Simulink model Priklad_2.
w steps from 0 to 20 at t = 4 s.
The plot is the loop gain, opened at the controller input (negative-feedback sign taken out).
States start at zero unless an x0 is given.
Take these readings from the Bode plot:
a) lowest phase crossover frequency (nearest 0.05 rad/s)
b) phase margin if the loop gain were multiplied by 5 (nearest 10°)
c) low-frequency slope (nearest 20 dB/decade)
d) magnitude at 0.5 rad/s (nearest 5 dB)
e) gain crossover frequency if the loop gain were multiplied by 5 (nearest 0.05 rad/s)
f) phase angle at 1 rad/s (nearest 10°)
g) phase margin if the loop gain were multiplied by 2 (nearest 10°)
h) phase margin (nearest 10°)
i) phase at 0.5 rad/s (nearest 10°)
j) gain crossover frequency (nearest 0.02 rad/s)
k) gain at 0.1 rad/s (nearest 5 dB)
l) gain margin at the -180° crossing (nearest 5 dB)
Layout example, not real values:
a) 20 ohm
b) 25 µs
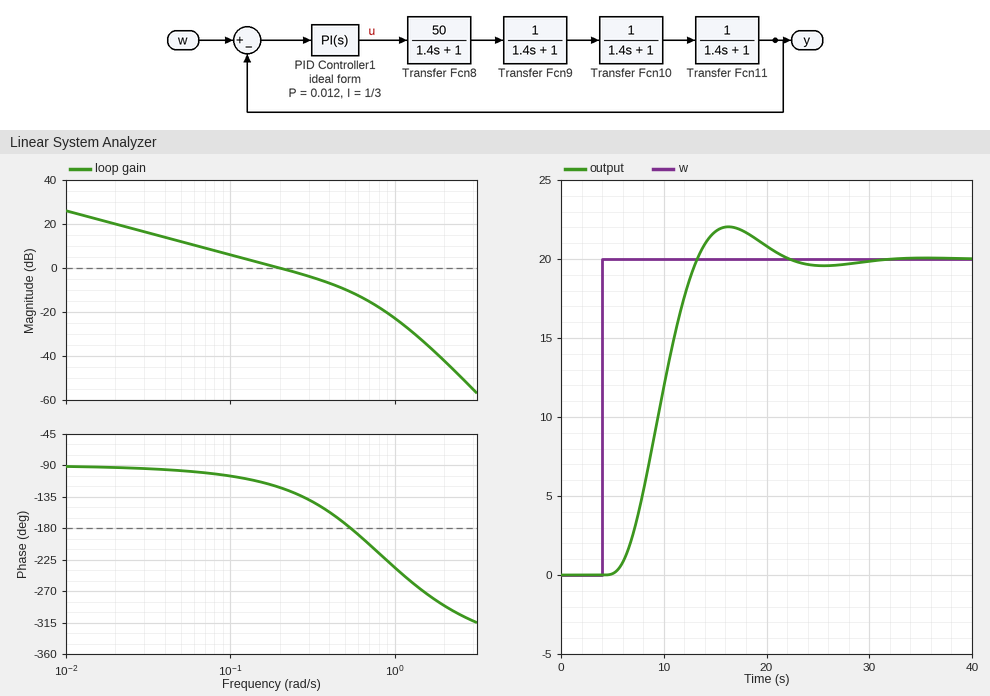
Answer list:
a) 0.55 rad/s
b) -20°
c) -20 dB/decade
d) -10 dB
e) 0.65 rad/s
f) -240°
g) 30°
h) 60°
i) -170°
j) 0.20 rad/s
k) 5 dB
l) 10 dB
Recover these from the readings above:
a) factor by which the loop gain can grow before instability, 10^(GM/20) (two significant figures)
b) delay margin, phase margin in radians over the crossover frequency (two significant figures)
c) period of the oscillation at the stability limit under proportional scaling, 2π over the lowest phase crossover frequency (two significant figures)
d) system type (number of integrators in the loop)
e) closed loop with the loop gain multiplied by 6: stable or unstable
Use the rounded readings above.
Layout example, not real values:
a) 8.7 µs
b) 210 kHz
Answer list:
a) 3.2
b) 5.2 s
c) 11 s
d) 1
e) unstable
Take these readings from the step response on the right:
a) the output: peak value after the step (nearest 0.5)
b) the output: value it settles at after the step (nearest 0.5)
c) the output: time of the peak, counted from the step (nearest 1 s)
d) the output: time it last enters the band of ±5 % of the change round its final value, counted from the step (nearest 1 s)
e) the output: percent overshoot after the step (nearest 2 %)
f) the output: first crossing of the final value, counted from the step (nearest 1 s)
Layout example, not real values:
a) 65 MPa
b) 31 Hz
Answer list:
a) 22.0
b) 20.0
c) 12 s
d) 16 s
e) 10 %
f) 9 s
